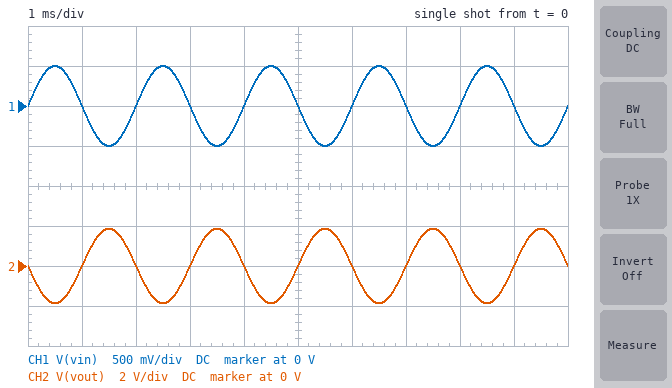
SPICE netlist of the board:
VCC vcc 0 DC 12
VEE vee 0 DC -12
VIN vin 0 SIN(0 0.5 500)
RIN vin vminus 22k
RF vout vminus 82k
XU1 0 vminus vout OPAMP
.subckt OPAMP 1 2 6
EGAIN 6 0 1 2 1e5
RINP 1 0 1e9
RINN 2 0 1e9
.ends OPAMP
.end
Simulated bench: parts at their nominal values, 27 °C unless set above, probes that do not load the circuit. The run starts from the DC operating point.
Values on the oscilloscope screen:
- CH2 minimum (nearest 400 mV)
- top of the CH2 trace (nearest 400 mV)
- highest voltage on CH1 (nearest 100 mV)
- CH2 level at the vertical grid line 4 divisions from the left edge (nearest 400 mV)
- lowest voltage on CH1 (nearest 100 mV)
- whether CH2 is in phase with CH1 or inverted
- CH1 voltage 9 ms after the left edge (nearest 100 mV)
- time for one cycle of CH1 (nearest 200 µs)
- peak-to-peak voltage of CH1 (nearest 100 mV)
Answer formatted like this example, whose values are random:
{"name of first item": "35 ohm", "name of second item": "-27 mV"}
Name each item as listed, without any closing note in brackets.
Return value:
{"CH2 minimum": "-2.0 V", "top of the CH2 trace": "2.0 V", "highest voltage on CH1": "500 mV", "CH2 level at the vertical grid line 4 divisions from the left edge": "0 V", "lowest voltage on CH1": "-500 mV", "whether CH2 is in phase with CH1 or inverted": "inverted", "CH1 voltage 9 ms after the left edge": "0 V", "time for one cycle of CH1": "2.0 ms", "peak-to-peak voltage of CH1": "1.0 V"}
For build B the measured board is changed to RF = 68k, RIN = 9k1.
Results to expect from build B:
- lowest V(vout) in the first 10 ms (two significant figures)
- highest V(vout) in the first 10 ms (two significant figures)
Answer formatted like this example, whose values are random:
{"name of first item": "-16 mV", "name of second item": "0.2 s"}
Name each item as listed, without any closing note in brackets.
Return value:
{"lowest V(vout) in the first 10 ms": "-3.7 V", "highest V(vout) in the first 10 ms": "3.7 V"}
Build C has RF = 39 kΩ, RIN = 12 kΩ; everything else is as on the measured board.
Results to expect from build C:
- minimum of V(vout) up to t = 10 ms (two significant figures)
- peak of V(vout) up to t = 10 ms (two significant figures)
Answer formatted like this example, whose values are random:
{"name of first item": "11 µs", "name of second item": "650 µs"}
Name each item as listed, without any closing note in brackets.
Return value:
{"minimum of V(vout) up to t = 10 ms": "-1.6 V", "peak of V(vout) up to t = 10 ms": "1.6 V"}
